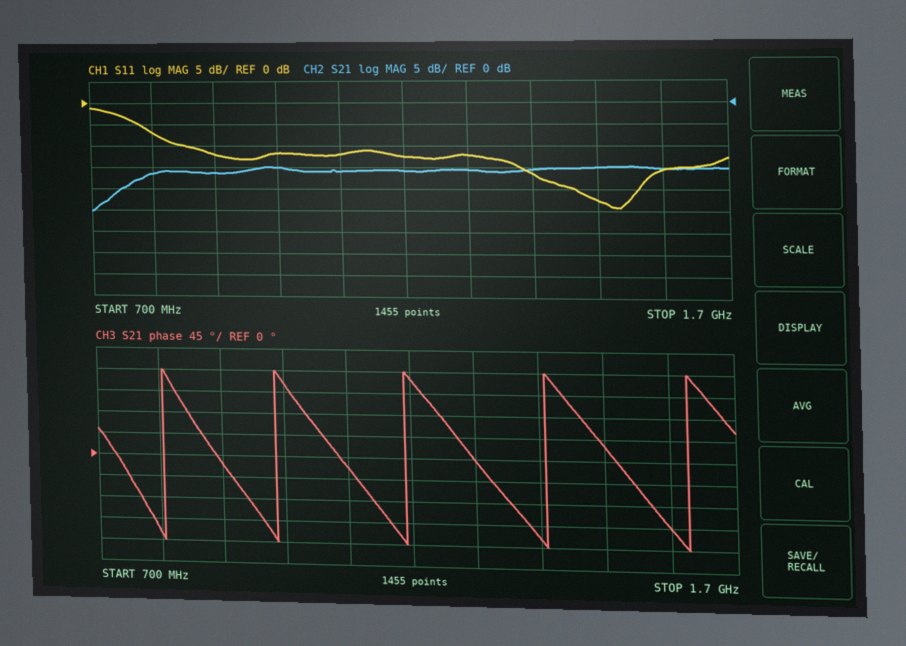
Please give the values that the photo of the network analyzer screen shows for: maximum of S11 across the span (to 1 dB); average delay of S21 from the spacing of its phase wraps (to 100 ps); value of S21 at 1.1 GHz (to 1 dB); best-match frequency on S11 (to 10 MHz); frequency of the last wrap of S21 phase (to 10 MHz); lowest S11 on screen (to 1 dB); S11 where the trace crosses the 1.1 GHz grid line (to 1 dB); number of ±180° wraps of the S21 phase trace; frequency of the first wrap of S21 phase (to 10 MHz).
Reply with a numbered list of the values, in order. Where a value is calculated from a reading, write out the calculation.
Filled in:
1. -1 dB
2. 4 cycles / (1.63 GHz − 810 MHz) ≈ 4.9 ns
3. -16 dB
4. 1.53 GHz
5. 1.63 GHz
6. -24 dB
7. -12 dB
8. 5
9. 810 MHz
